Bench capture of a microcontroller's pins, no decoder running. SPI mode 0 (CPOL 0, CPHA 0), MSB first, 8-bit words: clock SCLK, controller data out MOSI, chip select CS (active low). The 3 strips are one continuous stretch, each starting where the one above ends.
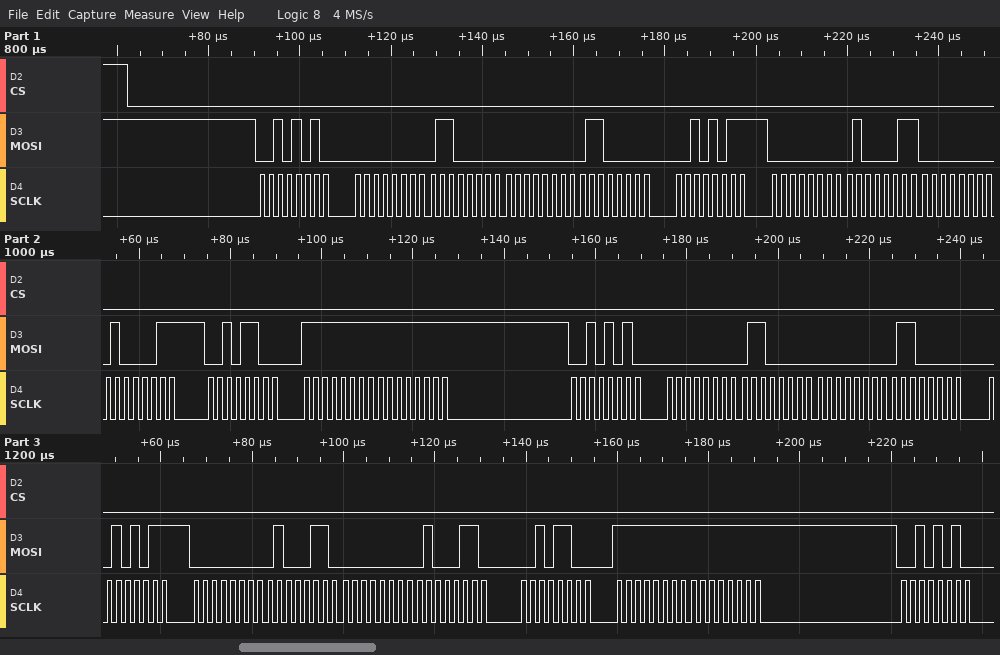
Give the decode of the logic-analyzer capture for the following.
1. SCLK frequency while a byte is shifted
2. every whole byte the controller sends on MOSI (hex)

500 kHz
2A 00 60 00 60 2B 00 43 00 43 2C FF FF 2A 00 60 00 60 2B 00 46 00 46 2C FF FF 2A
